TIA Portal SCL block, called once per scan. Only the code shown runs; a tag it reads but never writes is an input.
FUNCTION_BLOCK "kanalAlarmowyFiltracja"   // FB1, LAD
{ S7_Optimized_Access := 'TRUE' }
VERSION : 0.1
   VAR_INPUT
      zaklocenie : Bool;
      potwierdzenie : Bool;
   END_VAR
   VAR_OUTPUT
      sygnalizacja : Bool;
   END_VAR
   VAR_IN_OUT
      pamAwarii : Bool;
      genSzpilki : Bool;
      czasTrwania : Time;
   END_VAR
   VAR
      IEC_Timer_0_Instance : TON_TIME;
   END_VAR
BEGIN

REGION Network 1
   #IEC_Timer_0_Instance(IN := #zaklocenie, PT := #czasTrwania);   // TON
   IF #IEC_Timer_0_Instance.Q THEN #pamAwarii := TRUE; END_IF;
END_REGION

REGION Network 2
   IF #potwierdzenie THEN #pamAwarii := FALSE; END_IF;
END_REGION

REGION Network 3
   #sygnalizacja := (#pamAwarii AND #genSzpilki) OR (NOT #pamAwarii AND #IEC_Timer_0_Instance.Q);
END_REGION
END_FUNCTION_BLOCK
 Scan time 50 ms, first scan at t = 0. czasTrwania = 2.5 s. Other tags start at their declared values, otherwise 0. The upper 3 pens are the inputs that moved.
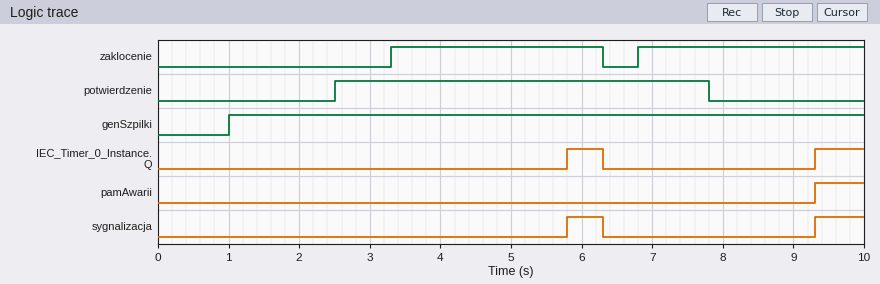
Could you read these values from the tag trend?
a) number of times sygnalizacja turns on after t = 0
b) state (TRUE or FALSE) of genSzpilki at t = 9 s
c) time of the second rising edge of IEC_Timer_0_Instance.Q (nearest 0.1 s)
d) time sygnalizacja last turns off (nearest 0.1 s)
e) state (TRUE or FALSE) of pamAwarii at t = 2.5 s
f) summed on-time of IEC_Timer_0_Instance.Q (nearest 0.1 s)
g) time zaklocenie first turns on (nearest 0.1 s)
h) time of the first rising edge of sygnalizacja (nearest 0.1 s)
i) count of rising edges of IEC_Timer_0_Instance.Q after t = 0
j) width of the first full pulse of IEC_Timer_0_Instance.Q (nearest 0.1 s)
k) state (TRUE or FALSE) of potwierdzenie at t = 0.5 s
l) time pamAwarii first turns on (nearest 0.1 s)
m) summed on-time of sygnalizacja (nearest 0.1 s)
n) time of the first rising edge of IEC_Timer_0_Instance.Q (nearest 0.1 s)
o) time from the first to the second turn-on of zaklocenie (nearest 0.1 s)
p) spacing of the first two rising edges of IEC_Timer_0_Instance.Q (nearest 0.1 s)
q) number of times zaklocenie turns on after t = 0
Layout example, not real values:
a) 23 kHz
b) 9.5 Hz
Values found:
a) 2
b) TRUE
c) 9.3 s
d) 6.3 s
e) FALSE
f) 1.2 s
g) 3.3 s
h) 5.8 s
i) 2
j) 0.5 s
k) FALSE
l) 9.3 s
m) 1.2 s
n) 5.8 s
o) 3.5 s
p) 3.5 s
q) 2
